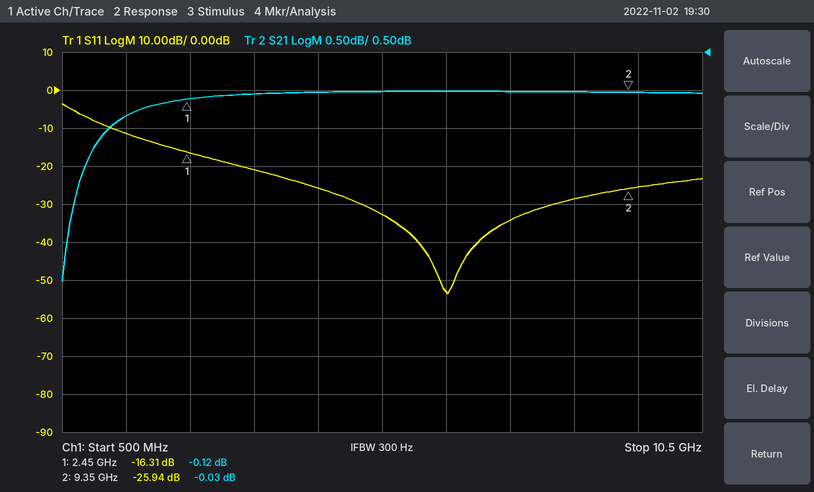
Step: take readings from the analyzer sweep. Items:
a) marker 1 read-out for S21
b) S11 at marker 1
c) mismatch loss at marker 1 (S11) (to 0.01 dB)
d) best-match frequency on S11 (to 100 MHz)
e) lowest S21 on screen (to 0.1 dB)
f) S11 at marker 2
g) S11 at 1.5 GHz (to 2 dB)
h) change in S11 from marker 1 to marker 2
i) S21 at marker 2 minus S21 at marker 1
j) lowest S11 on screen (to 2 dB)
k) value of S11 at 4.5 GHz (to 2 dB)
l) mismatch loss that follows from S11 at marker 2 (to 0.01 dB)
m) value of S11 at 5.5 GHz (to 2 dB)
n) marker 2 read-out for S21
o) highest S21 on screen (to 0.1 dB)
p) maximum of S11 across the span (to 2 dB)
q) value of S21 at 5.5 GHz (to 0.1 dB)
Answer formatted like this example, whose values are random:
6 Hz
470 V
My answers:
-0.12 dB
-16.31 dB
0.10 dB
6.5 GHz
-2.5 dB
-25.94 dB
-12 dB
-9.63 dB
0.09 dB
-54 dB
-26 dB
0.01 dB
-32 dB
-0.03 dB
0.0 dB
-4 dB
0.0 dB
